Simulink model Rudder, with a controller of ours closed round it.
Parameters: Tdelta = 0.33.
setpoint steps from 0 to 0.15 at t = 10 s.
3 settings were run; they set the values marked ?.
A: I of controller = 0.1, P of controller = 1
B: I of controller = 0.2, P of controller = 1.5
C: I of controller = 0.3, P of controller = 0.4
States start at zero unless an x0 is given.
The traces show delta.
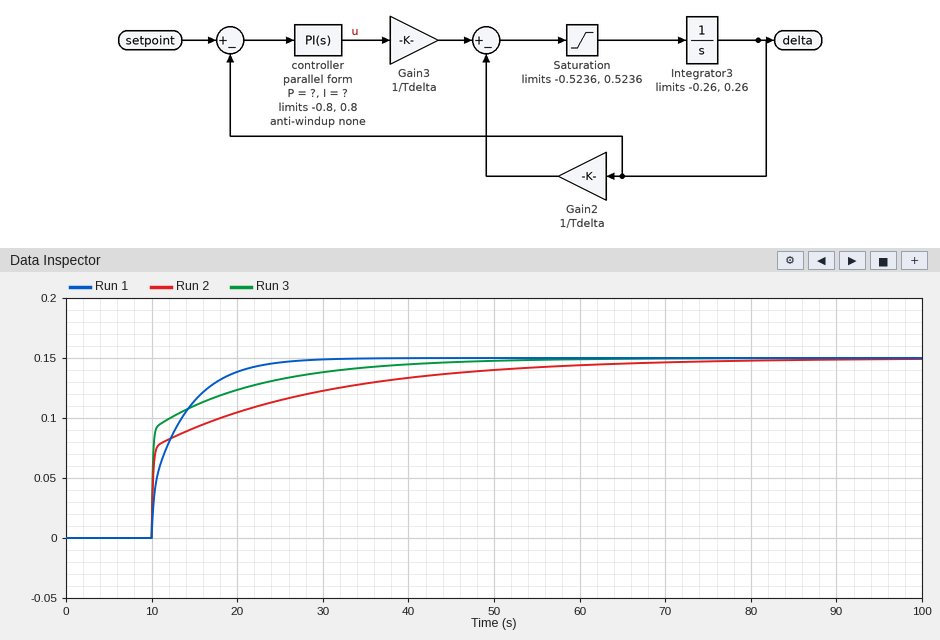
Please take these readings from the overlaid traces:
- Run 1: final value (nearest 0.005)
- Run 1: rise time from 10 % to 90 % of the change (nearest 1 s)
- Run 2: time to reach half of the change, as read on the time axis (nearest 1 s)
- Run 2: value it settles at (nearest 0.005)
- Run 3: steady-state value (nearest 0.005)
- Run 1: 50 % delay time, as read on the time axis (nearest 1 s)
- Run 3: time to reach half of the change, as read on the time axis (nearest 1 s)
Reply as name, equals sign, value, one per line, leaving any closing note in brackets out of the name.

Run 1: final value = 0.150
Run 1: rise time from 10 % to 90 % of the change = 9 s
Run 2: time to reach half of the change, as read on the time axis = 11 s
Run 2: value it settles at = 0.150
Run 3: steady-state value = 0.150
Run 1: 50 % delay time, as read on the time axis = 12 s
Run 3: time to reach half of the change, as read on the time axis = 10 s
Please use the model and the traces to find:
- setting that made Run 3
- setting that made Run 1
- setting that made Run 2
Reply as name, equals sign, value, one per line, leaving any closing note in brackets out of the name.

setting that made Run 3 = B
setting that made Run 1 = C
setting that made Run 2 = A
